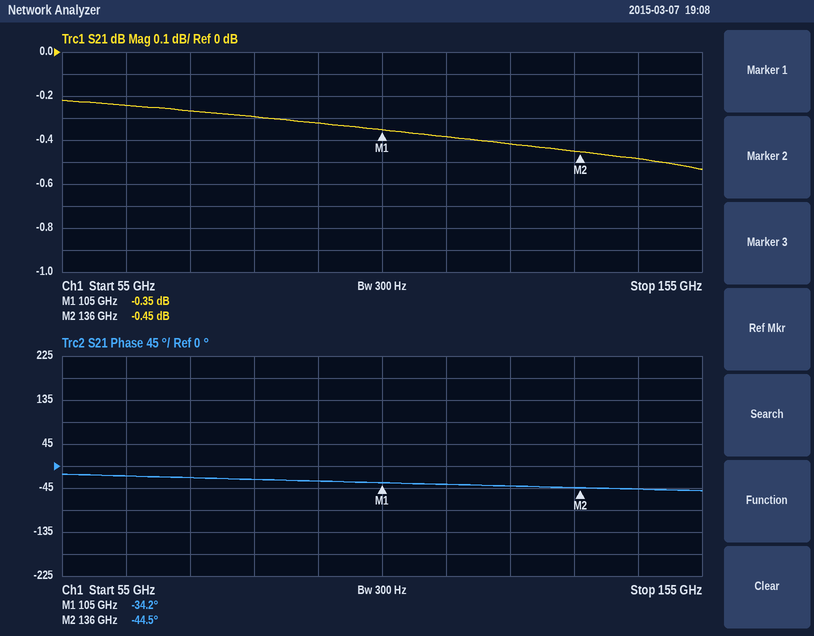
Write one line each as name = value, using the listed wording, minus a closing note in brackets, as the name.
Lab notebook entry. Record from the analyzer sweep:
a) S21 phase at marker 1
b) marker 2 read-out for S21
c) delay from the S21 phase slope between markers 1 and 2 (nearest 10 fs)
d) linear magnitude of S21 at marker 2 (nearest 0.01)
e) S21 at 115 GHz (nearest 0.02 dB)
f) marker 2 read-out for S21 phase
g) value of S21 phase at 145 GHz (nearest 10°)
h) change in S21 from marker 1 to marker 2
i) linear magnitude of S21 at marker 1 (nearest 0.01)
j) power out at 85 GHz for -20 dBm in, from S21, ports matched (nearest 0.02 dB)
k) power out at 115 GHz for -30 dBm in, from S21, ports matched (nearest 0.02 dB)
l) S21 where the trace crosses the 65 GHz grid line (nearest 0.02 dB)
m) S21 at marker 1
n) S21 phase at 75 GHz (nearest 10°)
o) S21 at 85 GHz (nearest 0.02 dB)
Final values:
S21 phase at marker 1 = -34.2°
marker 2 read-out for S21 = -0.45 dB
delay from the S21 phase slope between markers 1 and 2 = 920 fs
linear magnitude of S21 at marker 2 = 0.95
S21 at 115 GHz = -0.38 dB
marker 2 read-out for S21 phase = -44.5°
value of S21 phase at 145 GHz = -50°
change in S21 from marker 1 to marker 2 = -0.10 dB
linear magnitude of S21 at marker 1 = 0.96
power out at 85 GHz for -20 dBm in, from S21, ports matched = -20.30 dBm
power out at 115 GHz for -30 dBm in, from S21, ports matched = -30.38 dBm
S21 where the trace crosses the 65 GHz grid line = -0.24 dB
S21 at marker 1 = -0.35 dB
S21 phase at 75 GHz = -20°
S21 at 85 GHz = -0.30 dB
